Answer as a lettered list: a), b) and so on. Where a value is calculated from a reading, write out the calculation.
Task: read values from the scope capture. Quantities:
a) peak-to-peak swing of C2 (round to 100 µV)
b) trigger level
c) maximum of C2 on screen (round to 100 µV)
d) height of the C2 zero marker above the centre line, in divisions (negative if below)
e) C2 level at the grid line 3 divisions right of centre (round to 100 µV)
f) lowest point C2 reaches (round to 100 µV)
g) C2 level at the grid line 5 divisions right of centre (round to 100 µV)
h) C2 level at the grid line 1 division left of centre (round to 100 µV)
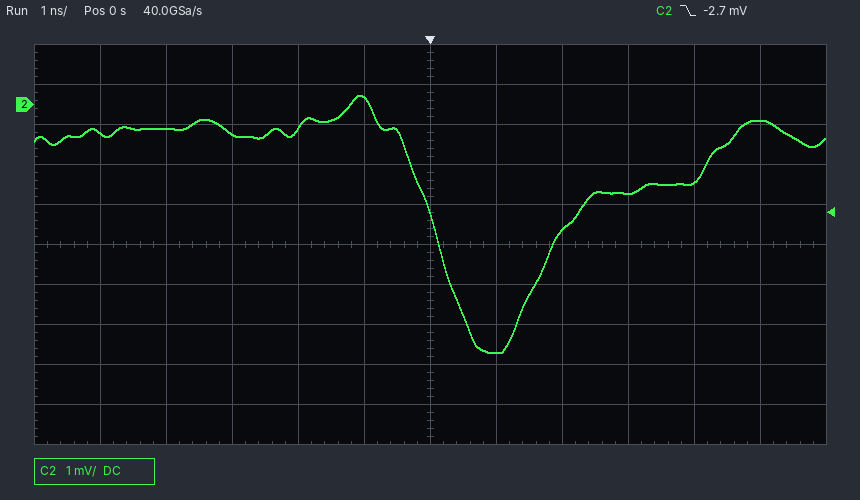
a) 200 µV − (-6.2 mV) = 6.4 mV
b) -2.7 mV
c) 200 µV
d) +3.5 div
e) -2.2 mV
f) -6.2 mV
g) -400 µV
h) 200 µV
